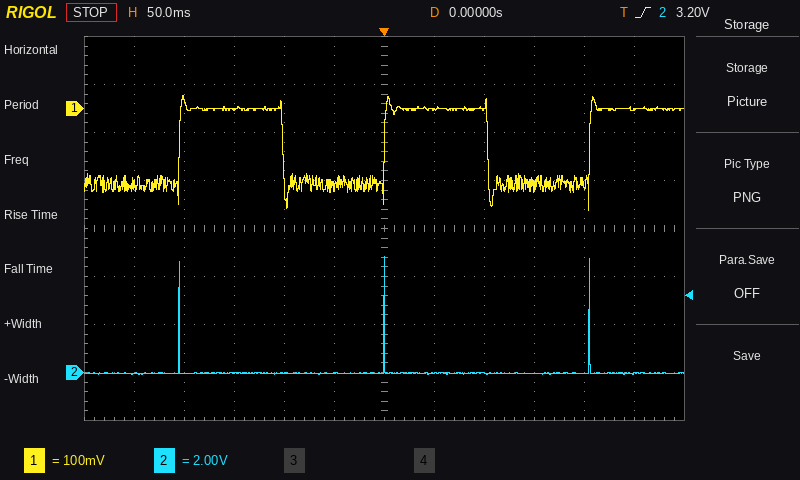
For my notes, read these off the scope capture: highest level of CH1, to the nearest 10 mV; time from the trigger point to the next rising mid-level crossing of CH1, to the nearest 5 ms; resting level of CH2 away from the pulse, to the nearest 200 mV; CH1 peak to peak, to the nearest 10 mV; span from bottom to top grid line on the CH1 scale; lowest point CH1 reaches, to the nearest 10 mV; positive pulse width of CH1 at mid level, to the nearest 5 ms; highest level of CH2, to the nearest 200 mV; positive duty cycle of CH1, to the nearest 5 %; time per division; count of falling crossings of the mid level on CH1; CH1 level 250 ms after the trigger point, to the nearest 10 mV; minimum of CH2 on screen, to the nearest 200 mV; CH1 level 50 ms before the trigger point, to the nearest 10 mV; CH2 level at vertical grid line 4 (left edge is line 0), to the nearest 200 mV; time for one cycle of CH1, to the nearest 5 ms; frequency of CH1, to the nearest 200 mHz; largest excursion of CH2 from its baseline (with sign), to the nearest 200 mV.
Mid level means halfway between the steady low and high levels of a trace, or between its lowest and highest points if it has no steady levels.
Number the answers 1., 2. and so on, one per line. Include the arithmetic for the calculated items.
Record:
1. 30 mV
2. 205 ms
3. 0.0 V
4. 30 mV − (-210 mV) = 240 mV
5. 800 mV
6. -210 mV
7. 105 ms
8. 4.8 V
9. 105 ms / 205 ms ≈ 51.2 %, so 50 % to the nearest 5 %
10. 50 ms
11. 2
12. 0 mV
13. 0.0 V
14. -160 mV
15. 0.0 V
16. 205 ms
17. 1 / 205 ms ≈ 4.88 Hz, so 4.8 Hz to the nearest 200 mHz
18. 4.8 V − (0.0 V) = +4.8 V
